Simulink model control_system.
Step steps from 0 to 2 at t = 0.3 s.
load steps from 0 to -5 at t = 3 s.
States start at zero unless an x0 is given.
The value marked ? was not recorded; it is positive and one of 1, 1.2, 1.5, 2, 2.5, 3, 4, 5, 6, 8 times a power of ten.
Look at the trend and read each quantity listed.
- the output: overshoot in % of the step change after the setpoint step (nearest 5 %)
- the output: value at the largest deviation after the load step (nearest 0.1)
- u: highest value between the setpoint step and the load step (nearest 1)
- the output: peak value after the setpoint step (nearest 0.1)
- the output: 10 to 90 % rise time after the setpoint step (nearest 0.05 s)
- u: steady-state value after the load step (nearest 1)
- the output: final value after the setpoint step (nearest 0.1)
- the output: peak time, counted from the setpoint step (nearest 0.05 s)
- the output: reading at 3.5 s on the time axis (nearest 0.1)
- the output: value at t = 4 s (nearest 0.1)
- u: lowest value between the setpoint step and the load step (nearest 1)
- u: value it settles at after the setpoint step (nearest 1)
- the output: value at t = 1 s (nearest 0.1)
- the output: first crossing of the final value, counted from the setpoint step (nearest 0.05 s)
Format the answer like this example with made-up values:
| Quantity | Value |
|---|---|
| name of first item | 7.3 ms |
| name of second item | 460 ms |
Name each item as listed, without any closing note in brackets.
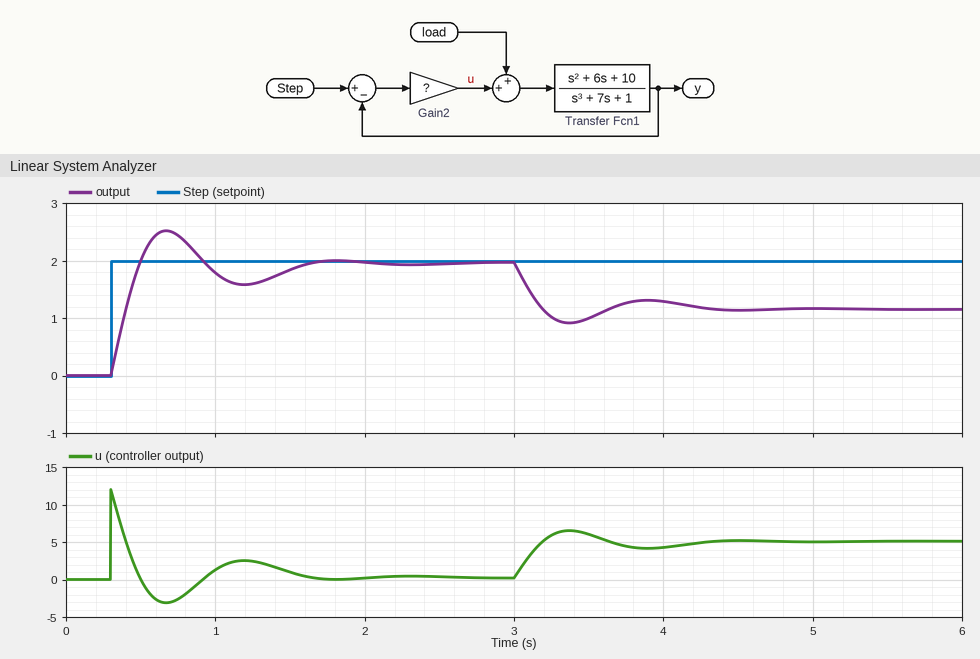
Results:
| Quantity | Value |
|---|---|
| the output: overshoot in % of the step change after the setpoint step | 30 % |
| the output: value at the largest deviation after the load step | 0.9 |
| u: highest value between the setpoint step and the load step | 12 |
| the output: peak value after the setpoint step | 2.5 |
| the output: 10 to 90 % rise time after the setpoint step | 0.15 s |
| u: steady-state value after the load step | 5 |
| the output: final value after the setpoint step | 2.0 |
| the output: peak time, counted from the setpoint step | 0.35 s |
| the output: reading at 3.5 s on the time axis | 1.0 |
| the output: value at t = 4 s | 1.3 |
| u: lowest value between the setpoint step and the load step | -3 |
| u: value it settles at after the setpoint step | 0 |
| the output: value at t = 1 s | 1.8 |
| the output: first crossing of the final value, counted from the setpoint step | 0.20 s |
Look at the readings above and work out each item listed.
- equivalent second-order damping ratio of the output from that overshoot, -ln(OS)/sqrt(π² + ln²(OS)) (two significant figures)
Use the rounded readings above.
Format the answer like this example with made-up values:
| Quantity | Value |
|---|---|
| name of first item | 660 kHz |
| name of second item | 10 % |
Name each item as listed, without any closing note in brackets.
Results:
| Quantity | Value |
|---|---|
| equivalent second-order damping ratio of the output from that overshoot, -ln(OS)/sqrt(π² + ln²(OS)) | 0.36 |
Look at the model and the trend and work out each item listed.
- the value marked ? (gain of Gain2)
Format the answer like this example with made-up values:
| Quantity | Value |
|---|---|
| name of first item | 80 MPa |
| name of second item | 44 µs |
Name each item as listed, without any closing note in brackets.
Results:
| Quantity | Value |
|---|---|
| the value marked ? | 6 |
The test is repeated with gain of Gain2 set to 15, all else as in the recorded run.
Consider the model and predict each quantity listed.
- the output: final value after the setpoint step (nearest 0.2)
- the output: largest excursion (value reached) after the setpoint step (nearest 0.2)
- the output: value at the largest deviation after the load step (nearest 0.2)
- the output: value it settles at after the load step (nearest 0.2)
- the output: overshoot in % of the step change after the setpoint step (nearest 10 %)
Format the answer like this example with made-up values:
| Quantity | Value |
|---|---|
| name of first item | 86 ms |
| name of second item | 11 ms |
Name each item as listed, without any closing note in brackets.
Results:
| Quantity | Value |
|---|---|
| the output: final value after the setpoint step | 2.0 |
| the output: largest excursion (value reached) after the setpoint step | 2.4 |
| the output: value at the largest deviation after the load step | 1.6 |
| the output: value it settles at after the load step | 1.6 |
| the output: overshoot in % of the step change after the setpoint step | 20 % |
